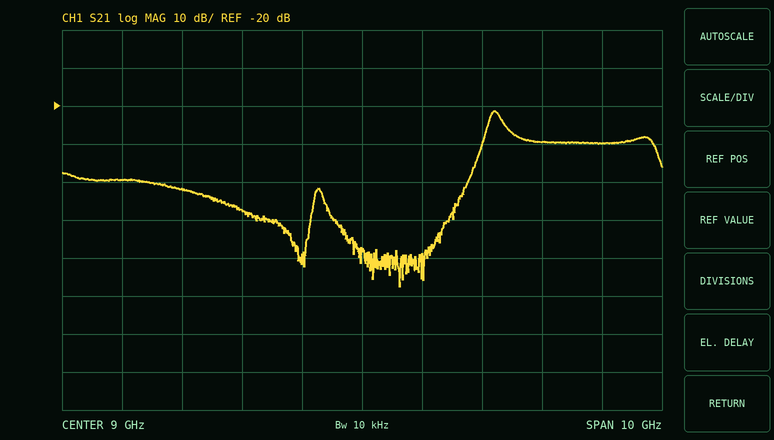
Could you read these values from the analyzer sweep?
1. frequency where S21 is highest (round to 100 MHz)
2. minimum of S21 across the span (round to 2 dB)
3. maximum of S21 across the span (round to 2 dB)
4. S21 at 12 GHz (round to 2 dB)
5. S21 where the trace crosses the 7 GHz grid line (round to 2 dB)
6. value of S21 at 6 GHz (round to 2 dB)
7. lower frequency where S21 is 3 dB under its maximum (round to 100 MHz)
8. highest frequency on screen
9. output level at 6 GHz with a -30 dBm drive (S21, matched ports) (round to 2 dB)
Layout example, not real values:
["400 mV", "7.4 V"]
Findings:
["11.2 GHz", "-68 dB", "-22 dB", "-30 dB", "-48 dB", "-42 dB", "11.1 GHz", "14 GHz", "-72 dBm"]
